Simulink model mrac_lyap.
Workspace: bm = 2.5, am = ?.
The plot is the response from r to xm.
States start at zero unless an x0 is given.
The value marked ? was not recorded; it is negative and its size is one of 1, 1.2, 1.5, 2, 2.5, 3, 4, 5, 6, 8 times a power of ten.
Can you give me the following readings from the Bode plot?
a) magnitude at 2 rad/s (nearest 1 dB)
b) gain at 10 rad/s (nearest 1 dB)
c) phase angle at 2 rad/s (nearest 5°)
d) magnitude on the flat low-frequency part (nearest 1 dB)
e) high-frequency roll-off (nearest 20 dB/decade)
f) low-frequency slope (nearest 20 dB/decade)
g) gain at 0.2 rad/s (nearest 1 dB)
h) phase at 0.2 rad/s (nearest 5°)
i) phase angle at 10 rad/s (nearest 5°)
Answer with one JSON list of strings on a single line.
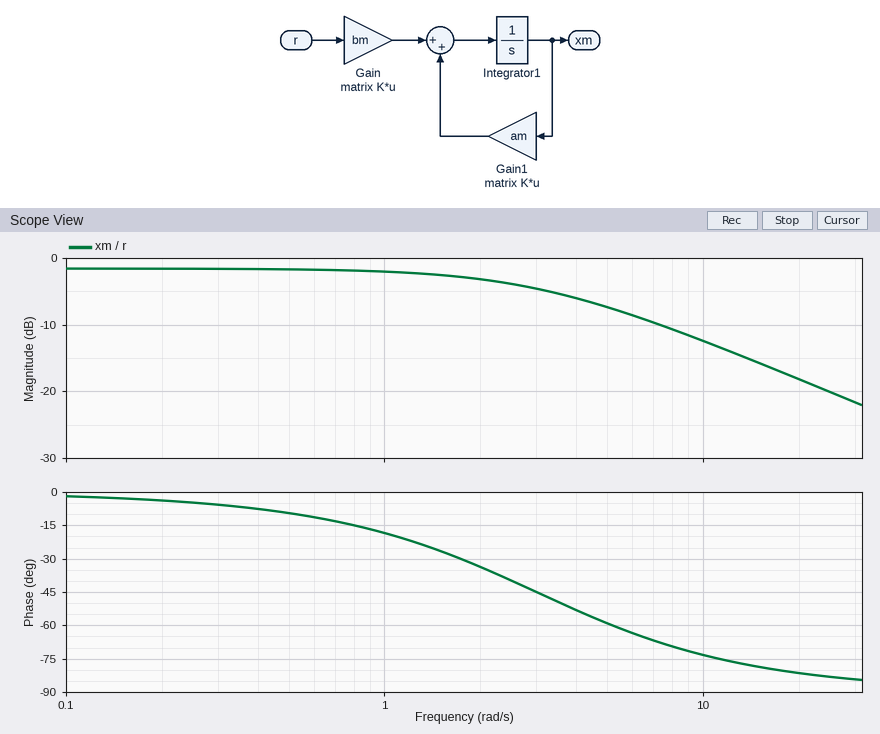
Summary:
["-3 dB", "-12 dB", "-35°", "-2 dB", "-20 dB/decade", "0 dB/decade", "-2 dB", "-5°", "-75°"]
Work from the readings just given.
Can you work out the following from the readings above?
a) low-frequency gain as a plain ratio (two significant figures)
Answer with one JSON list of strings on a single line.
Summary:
["0.79"]
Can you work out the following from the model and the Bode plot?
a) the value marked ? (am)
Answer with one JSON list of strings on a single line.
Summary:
["-3"]
